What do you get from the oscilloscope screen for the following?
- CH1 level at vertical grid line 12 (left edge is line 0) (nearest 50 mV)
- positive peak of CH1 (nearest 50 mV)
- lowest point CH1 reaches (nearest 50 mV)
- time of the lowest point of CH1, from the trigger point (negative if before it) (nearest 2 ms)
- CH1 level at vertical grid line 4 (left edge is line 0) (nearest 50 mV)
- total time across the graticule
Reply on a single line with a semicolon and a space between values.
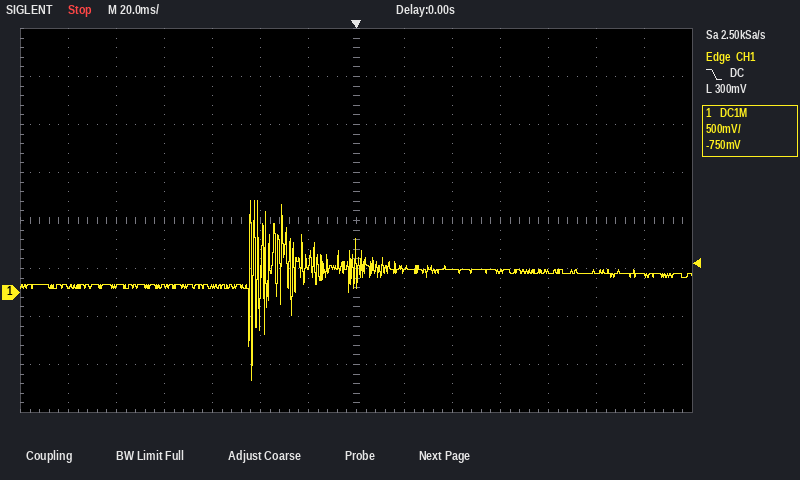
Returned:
200 mV; 950 mV; -900 mV; -44 ms; 50 mV; 280 ms
